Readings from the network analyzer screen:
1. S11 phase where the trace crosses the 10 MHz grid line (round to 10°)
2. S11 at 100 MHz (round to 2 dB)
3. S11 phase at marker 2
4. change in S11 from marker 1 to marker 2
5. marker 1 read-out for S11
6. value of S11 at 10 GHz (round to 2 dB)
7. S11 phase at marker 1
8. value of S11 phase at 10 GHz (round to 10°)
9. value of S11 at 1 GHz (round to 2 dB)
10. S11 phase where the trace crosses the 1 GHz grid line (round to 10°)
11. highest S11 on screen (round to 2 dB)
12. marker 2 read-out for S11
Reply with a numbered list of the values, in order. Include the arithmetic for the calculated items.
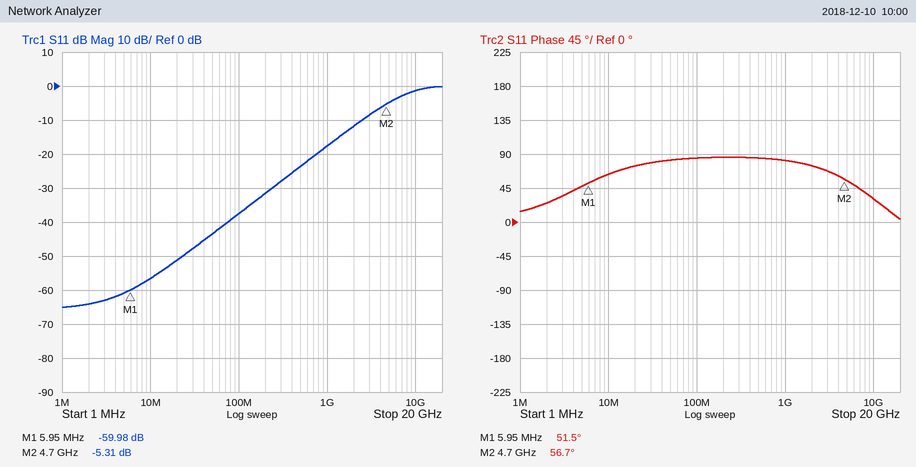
1. 60°
2. -38 dB
3. 56.7°
4. -5.31 − (-59.98) = 54.67 dB
5. -59.98 dB
6. -2 dB
7. 51.5°
8. 30°
9. -18 dB
10. 80°
11. 0 dB
12. -5.31 dB
